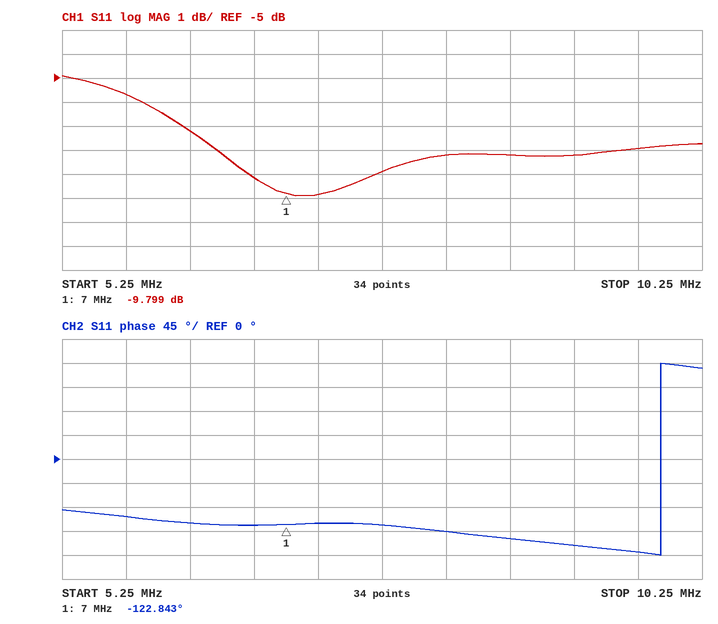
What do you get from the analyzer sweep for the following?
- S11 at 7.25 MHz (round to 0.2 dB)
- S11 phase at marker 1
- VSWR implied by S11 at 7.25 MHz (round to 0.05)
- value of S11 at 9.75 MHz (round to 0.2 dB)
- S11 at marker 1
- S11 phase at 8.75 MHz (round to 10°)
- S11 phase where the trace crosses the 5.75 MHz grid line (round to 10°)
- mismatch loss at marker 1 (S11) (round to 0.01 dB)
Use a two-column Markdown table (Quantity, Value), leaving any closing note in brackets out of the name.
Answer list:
| Quantity | Value |
|---|---|
| S11 at 7.25 MHz | -9.8 dB |
| S11 phase at marker 1 | -122.843° |
| VSWR implied by S11 at 7.25 MHz | 1.95 |
| value of S11 at 9.75 MHz | -8.0 dB |
| S11 at marker 1 | -9.799 dB |
| S11 phase at 8.75 MHz | -150° |
| S11 phase where the trace crosses the 5.75 MHz grid line | -110° |
| mismatch loss at marker 1 (S11) | 0.48 dB |
